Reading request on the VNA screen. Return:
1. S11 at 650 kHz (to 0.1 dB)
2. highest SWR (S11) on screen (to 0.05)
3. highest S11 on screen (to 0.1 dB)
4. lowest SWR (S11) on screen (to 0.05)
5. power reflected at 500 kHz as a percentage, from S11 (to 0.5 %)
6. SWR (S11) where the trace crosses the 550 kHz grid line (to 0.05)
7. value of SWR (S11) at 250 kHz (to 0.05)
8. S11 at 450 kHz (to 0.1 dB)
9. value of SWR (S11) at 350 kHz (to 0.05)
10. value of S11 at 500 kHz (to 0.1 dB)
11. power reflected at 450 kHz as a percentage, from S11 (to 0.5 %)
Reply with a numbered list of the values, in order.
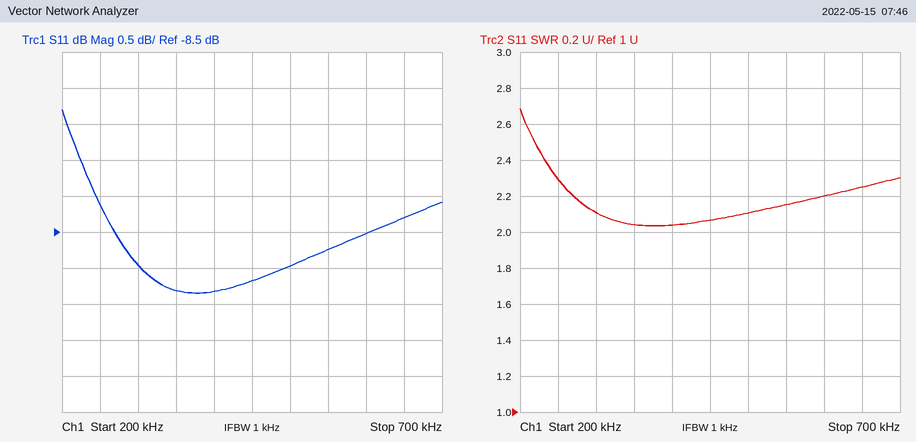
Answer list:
1. -8.3 dB
2. 2.70
3. -6.8 dB
4. 2.05
5. 12.5 %
6. 2.15
7. 2.30
8. -9.2 dB
9. 2.05
10. -9.0 dB
11. 12.0 %
